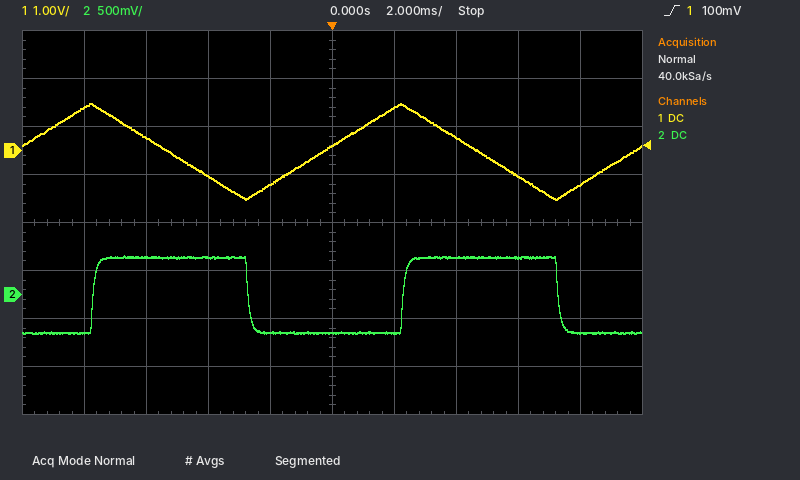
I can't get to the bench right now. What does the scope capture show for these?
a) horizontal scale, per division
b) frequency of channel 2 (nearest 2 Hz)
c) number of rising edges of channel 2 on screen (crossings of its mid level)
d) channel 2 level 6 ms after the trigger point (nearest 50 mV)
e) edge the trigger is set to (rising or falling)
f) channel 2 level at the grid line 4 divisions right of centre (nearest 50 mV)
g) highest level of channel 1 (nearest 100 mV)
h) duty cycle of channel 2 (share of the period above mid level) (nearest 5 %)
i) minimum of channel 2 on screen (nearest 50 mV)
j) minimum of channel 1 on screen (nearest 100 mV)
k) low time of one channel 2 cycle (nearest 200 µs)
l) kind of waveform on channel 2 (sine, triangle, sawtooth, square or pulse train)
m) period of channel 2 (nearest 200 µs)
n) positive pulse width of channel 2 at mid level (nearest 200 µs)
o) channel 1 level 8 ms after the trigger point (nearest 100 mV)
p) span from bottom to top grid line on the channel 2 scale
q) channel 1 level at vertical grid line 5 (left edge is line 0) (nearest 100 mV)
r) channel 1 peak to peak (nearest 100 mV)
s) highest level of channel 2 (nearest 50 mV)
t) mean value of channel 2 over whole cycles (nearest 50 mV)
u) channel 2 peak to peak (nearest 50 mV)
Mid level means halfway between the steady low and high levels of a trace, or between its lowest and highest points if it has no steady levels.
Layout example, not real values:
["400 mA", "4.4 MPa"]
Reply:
["2 ms", "100 Hz", "2", "400 mV", "rising", "-400 mV", "1.0 V", "50 %", "-400 mV", "-1.0 V", "5.0 ms", "square", "10.0 ms", "5.0 ms", "-700 mV", "4 V", "100 mV", "2.0 V", "400 mV", "0 mV", "800 mV"]
